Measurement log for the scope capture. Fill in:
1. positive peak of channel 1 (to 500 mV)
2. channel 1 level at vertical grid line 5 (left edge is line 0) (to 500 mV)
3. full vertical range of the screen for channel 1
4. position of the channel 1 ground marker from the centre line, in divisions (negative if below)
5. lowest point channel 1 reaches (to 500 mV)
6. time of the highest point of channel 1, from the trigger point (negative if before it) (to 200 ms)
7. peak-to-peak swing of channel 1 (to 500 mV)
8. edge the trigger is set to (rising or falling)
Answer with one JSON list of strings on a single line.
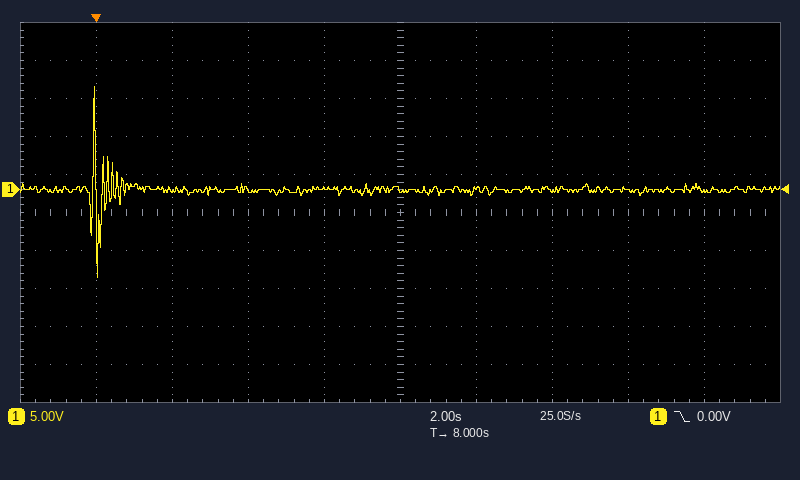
["13.5 V", "0.0 V", "50 V", "+0.6 div", "-11.5 V", "0.0 s", "25.0 V", "falling"]
